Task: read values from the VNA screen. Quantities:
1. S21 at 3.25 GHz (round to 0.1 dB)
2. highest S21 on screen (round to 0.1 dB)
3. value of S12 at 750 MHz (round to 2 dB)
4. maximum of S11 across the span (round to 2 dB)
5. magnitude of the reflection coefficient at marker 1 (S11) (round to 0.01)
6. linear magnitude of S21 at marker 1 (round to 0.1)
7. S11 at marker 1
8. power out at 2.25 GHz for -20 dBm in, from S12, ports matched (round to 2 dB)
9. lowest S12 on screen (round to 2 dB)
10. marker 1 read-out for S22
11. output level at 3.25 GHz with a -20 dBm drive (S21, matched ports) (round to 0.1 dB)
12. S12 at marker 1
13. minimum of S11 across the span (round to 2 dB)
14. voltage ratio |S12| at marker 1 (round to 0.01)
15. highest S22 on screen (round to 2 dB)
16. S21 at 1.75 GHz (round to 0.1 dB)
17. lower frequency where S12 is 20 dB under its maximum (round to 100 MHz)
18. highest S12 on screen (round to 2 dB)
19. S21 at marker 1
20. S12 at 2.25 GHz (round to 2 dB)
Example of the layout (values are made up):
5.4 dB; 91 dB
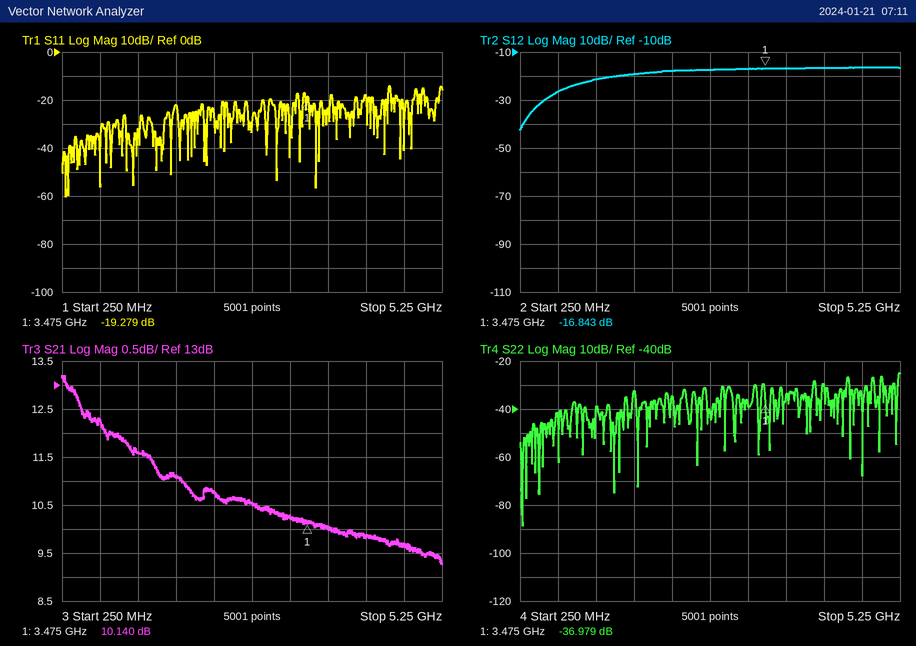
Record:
10.2 dB; 13.2 dB; -26 dB; -14 dB; 0.11; 3.2; -19.279 dB; -38 dBm; -42 dB; -36.979 dB; -9.8 dBm; -16.843 dB; -60 dB; 0.14; -24 dB; 11.1 dB; 400 MHz; -16 dB; 10.140 dB; -18 dB
